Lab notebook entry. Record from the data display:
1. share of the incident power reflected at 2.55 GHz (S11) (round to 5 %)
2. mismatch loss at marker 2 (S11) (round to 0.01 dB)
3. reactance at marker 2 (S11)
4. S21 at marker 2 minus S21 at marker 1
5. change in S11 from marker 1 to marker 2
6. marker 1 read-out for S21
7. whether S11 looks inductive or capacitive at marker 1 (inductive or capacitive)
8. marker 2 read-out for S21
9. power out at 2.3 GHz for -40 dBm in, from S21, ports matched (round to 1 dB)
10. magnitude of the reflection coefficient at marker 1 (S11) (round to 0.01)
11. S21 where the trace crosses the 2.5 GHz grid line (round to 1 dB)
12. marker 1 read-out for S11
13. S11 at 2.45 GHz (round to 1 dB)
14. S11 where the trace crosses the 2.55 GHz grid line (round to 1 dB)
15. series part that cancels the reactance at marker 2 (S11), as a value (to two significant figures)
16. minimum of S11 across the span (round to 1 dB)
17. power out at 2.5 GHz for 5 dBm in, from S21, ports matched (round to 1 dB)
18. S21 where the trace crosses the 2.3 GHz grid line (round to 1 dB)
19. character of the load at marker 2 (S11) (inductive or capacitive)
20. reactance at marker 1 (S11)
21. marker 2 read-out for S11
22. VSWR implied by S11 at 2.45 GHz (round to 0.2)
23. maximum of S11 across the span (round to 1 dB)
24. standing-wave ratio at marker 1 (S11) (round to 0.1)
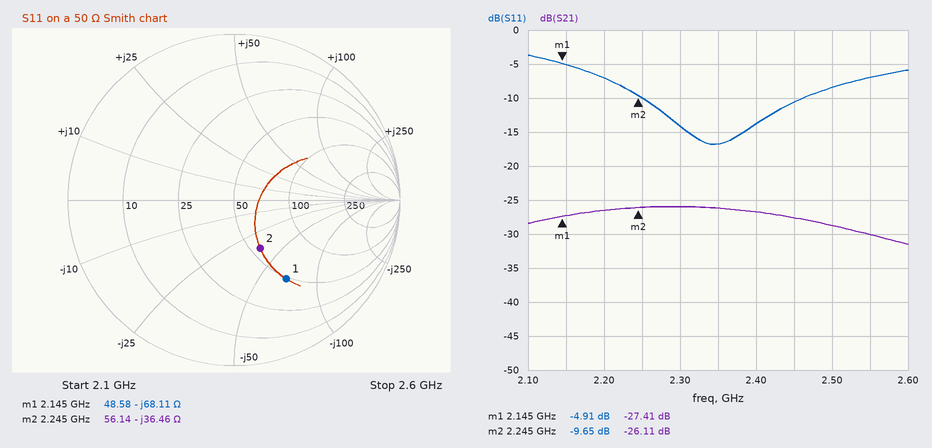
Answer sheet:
20 %
0.50 dB
-36.46 Ω
1.30 dB
-4.74 dB
-27.41 dB
capacitive
-26.11 dB
-66 dBm
0.57
-29 dB
-4.91 dB
-11 dB
-7 dB
2.6 nH
-17 dB
-24 dBm
-26 dB
capacitive
-68.11 Ω
-9.65 dB
1.8
-4 dB
3.6
